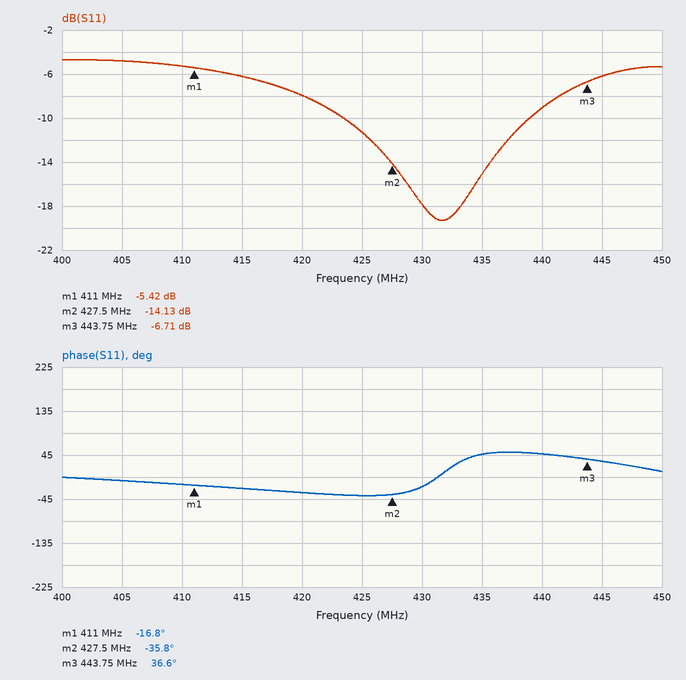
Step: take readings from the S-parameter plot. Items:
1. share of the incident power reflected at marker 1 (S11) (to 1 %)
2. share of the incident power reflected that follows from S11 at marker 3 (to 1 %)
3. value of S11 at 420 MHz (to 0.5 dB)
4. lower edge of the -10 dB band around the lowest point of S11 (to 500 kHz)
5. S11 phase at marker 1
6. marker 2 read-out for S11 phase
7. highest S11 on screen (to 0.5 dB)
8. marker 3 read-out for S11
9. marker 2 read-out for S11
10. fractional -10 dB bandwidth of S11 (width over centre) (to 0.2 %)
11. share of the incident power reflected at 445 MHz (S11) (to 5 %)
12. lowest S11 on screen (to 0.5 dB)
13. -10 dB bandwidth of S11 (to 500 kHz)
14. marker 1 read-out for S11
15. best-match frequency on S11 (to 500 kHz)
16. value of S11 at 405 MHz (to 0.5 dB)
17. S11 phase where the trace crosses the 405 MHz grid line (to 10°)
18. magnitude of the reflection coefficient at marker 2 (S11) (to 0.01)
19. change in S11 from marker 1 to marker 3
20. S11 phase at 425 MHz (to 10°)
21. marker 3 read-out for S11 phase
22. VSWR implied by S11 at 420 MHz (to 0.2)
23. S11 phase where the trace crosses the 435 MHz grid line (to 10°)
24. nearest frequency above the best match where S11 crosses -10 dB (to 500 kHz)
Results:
29 %
21 %
-8.0 dB
423.5 MHz
-16.8°
-35.8°
-4.5 dB
-6.71 dB
-14.13 dB
3.6 %
25 %
-19.5 dB
15.5 MHz
-5.42 dB
431.5 MHz
-5.0 dB
-10°
0.20
-1.29 dB
-40°
36.6°
2.4
50°
439.0 MHz
